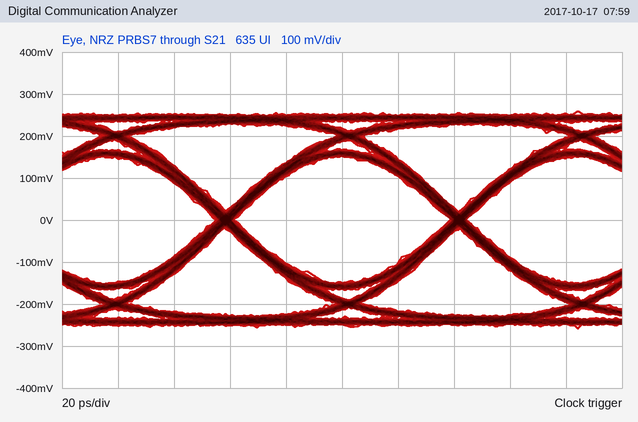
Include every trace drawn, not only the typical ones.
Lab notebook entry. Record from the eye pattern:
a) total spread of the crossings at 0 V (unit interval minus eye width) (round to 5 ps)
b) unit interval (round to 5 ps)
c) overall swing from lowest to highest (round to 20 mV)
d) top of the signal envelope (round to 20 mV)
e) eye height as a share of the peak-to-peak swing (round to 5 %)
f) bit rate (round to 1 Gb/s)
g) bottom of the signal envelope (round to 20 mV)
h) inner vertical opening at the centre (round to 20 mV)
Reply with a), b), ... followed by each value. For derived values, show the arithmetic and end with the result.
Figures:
a) 5 ps
b) 85 ps
c) 520 mV
d) 260 mV
e) 300 mV / 520 mV ≈ 57.7 %, so 60 % to the nearest 5 %
f) 12 Gb/s
g) -260 mV
h) 300 mV
